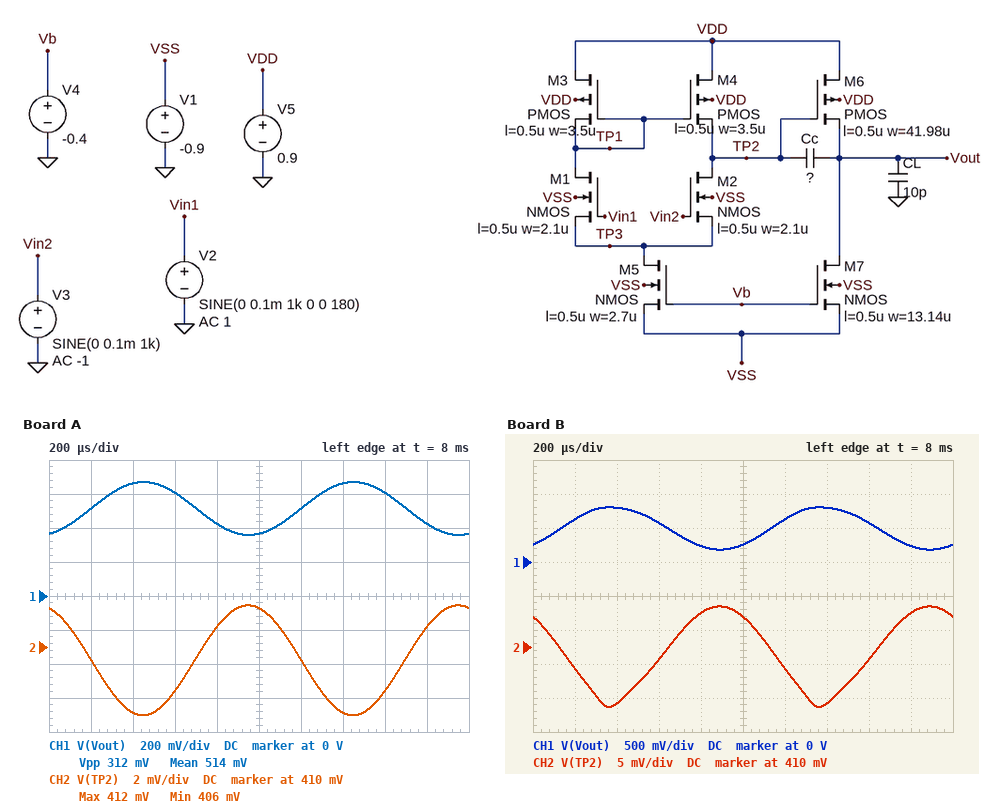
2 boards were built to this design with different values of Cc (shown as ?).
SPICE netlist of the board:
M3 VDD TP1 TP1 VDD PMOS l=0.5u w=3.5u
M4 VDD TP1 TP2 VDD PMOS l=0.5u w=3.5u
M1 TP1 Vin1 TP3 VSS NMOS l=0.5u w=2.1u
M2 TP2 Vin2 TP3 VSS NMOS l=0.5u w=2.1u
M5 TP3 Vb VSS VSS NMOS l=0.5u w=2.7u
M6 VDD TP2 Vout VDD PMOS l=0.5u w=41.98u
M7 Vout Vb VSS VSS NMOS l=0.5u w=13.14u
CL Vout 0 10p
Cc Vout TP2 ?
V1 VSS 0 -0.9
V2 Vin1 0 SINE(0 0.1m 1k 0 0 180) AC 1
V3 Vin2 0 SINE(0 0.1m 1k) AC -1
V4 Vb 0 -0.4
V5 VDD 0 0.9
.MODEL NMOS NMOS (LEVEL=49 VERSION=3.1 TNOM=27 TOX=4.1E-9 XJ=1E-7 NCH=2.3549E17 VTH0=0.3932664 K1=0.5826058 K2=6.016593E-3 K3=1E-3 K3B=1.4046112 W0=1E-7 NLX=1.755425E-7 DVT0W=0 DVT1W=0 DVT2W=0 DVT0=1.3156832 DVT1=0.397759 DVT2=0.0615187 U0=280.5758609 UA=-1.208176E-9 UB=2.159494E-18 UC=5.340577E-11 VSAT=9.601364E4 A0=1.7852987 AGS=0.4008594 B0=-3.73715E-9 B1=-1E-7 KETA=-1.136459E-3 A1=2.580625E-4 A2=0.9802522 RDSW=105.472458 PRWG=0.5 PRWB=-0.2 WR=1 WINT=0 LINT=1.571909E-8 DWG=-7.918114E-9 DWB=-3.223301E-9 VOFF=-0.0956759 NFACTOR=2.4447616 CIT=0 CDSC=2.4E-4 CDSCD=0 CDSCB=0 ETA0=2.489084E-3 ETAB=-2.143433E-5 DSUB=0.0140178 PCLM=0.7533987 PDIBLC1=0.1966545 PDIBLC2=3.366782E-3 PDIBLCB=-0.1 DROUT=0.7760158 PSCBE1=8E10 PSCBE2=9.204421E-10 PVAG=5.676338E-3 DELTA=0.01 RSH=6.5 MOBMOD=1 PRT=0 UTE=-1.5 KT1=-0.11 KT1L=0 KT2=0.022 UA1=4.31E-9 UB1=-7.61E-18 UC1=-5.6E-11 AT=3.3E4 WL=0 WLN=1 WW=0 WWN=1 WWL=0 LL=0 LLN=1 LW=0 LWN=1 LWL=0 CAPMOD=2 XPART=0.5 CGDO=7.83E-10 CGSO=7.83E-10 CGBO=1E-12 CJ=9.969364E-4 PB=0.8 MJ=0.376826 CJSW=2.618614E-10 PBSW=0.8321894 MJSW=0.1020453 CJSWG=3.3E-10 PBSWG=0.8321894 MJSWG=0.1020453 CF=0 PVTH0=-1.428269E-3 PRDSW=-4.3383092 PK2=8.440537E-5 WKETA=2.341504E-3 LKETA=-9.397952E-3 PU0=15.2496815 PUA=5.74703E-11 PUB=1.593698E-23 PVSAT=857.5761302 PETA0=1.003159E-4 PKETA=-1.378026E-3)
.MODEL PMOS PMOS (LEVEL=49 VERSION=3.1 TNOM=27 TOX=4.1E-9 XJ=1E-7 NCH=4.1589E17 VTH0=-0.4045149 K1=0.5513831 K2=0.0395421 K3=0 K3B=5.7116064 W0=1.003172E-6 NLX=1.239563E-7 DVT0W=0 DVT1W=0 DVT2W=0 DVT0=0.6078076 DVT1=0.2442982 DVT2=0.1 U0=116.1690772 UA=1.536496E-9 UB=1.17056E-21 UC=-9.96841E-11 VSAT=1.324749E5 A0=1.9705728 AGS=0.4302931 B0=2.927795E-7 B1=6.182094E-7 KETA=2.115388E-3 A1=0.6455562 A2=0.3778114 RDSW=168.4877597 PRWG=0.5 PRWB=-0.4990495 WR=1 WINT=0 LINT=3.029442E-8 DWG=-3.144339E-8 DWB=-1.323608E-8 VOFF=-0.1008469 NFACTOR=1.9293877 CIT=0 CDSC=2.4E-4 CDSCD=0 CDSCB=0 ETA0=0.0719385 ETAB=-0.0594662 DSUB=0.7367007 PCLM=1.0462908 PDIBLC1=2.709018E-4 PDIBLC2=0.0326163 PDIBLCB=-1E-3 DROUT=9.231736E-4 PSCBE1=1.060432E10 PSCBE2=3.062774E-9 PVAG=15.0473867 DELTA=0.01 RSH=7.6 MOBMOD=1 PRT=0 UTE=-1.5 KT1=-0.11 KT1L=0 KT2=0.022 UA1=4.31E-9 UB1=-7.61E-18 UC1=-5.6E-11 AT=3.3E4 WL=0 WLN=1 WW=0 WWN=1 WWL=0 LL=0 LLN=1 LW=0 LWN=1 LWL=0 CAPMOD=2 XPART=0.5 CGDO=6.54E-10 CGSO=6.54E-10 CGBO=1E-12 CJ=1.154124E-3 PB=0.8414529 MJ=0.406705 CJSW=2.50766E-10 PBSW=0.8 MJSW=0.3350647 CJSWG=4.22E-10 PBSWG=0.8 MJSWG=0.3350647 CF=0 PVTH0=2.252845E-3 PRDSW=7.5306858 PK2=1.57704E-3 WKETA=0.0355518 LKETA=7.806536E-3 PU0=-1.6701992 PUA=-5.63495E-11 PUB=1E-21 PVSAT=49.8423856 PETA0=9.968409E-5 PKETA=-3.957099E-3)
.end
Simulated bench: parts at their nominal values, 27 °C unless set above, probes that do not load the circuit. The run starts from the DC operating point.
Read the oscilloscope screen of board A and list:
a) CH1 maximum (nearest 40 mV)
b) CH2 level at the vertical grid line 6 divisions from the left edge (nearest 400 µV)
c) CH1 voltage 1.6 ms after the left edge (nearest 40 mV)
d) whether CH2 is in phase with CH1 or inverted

680 mV
409.2 mV
600 mV
inverted
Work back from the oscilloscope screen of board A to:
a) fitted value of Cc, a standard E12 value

3.9 pF
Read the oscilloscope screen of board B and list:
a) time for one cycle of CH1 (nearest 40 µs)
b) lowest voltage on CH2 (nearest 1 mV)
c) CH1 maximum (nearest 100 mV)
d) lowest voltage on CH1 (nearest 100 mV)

1.00 ms
401 mV
800 mV
200 mV
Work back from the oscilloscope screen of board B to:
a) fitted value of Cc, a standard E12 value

1.5 pF
